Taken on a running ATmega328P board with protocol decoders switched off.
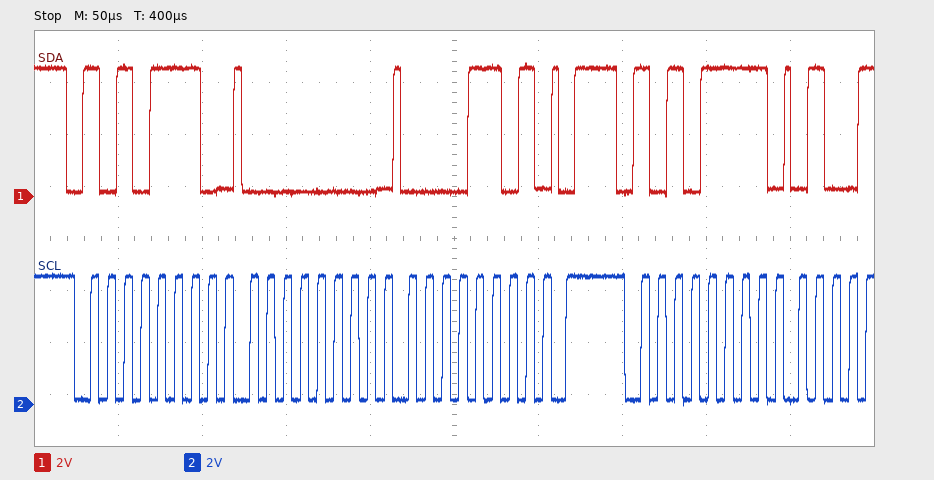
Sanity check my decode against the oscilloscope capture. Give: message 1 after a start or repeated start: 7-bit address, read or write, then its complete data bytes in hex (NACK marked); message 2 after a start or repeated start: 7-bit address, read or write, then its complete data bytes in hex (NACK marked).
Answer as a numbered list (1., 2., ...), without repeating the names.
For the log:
1. 0x57 write: 00 0D
2. 0x57 read
